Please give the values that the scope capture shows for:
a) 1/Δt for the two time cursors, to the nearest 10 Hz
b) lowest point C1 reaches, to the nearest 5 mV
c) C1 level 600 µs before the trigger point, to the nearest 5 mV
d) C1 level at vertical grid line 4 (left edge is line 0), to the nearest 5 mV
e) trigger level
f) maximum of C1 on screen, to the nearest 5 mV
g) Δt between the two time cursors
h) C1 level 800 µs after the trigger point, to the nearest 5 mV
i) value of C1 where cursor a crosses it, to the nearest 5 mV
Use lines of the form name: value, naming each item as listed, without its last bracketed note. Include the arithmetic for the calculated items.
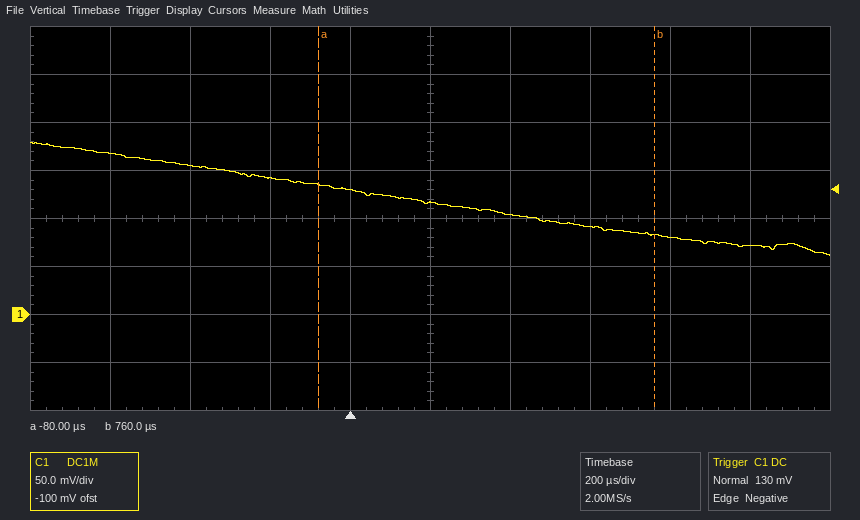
1/Δt for the two time cursors, to the nearest 10 Hz: 1 / 840 µs ≈ 1.19 kHz
lowest point C1 reaches, to the nearest 5 mV: 60 mV
C1 level 600 µs before the trigger point, to the nearest 5 mV: 170 mV
C1 level at vertical grid line 4 (left edge is line 0), to the nearest 5 mV: 130 mV
trigger level: 130 mV
maximum of C1 on screen, to the nearest 5 mV: 180 mV
Δt between the two time cursors: 760 µs − (-80 µs) = 840 µs
C1 level 800 µs after the trigger point, to the nearest 5 mV: 80 mV
value of C1 where cursor a crosses it, to the nearest 5 mV: 135 mV
